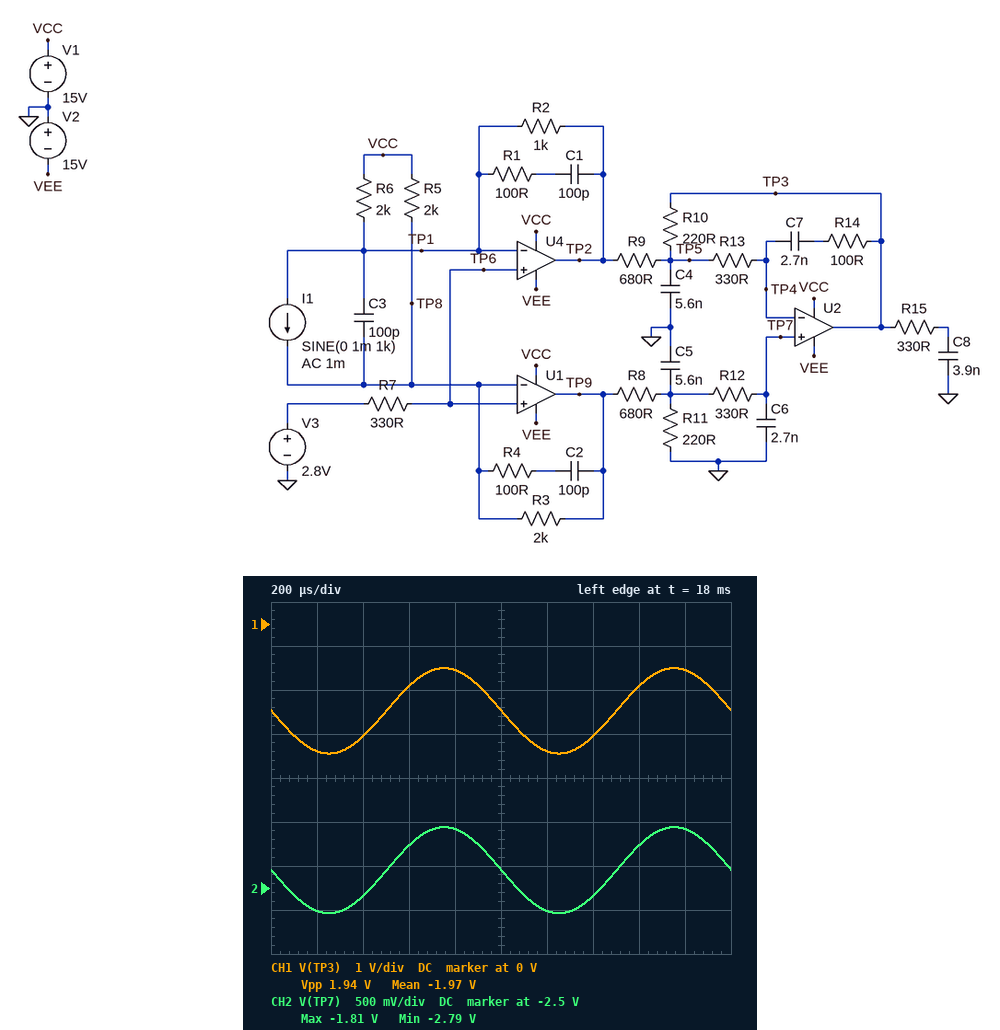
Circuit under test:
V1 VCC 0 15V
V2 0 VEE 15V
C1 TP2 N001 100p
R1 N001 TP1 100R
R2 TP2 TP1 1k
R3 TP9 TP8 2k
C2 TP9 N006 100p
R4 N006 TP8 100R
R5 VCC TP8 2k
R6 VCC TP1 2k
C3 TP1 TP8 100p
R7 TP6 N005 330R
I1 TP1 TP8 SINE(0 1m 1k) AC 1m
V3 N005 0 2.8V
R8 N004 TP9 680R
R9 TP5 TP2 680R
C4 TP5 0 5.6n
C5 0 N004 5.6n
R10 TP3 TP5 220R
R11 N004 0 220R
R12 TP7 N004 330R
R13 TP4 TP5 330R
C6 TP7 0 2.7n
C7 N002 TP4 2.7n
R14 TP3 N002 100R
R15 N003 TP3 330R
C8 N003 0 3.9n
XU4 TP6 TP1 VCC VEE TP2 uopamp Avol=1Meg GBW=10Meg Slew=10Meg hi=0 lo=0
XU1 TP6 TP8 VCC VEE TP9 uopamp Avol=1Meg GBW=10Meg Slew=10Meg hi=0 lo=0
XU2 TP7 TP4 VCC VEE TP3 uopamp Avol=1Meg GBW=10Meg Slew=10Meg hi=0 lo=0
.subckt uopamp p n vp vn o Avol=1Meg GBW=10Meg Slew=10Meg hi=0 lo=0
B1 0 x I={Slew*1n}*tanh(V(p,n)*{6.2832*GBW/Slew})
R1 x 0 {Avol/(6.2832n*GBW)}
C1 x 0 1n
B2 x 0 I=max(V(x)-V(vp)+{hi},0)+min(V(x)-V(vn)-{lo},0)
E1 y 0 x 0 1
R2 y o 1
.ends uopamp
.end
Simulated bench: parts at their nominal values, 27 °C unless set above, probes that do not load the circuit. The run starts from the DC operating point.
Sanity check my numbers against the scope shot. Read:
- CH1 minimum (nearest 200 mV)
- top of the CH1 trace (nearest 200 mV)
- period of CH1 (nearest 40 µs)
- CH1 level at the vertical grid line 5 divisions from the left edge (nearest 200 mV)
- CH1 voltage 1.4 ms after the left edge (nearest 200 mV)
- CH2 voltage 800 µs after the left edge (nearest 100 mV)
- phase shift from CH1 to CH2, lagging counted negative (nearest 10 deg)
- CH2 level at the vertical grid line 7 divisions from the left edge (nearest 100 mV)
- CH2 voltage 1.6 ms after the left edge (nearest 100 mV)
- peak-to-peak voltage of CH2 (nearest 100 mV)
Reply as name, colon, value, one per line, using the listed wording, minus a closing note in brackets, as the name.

CH1 minimum: -3.0 V
top of the CH1 trace: -1.0 V
period of CH1: 1.00 ms
CH1 level at the vertical grid line 5 divisions from the left edge: -2.0 V
CH1 voltage 1.4 ms after the left edge: -2.6 V
CH2 voltage 800 µs after the left edge: -1.8 V
phase shift from CH1 to CH2, lagging counted negative: 0 deg
CH2 level at the vertical grid line 7 divisions from the left edge: -2.6 V
CH2 voltage 1.6 ms after the left edge: -2.0 V
peak-to-peak voltage of CH2: 1.0 V
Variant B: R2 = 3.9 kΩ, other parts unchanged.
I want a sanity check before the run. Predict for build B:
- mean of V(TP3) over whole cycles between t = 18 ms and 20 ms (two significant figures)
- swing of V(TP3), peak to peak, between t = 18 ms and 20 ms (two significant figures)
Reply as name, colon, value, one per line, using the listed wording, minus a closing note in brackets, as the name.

mean of V(TP3) over whole cycles between t = 18 ms and 20 ms: 1.8 V
swing of V(TP3), peak to peak, between t = 18 ms and 20 ms: 1.3 V
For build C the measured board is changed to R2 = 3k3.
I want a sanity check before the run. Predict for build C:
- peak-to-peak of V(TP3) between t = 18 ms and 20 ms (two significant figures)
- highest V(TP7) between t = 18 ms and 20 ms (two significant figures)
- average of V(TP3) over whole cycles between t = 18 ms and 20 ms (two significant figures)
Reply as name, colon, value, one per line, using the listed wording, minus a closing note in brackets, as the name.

peak-to-peak of V(TP3) between t = 18 ms and 20 ms: 1.6 V
highest V(TP7) between t = 18 ms and 20 ms: -1.8 V
average of V(TP3) over whole cycles between t = 18 ms and 20 ms: 1.8 V
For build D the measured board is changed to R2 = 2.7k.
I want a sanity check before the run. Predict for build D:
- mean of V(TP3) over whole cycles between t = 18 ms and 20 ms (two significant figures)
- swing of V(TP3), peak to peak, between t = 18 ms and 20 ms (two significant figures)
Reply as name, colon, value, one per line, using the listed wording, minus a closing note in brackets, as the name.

mean of V(TP3) over whole cycles between t = 18 ms and 20 ms: 1.3 V
swing of V(TP3), peak to peak, between t = 18 ms and 20 ms: 2.6 V
